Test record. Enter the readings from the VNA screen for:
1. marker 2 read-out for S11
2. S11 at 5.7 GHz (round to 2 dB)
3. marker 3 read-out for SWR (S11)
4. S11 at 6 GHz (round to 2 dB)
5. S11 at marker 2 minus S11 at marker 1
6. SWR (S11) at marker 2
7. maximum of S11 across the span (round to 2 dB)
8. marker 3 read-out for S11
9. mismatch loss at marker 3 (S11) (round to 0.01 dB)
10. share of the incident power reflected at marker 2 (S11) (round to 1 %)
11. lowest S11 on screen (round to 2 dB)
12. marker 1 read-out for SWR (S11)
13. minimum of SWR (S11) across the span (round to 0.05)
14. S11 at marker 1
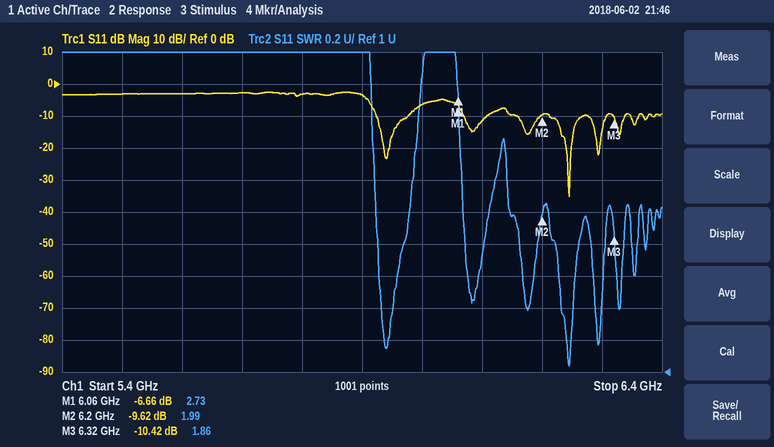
-9.62 dB
-2 dB
1.86
-6 dB
-2.96 dB
1.99
-2 dB
-10.42 dB
0.41 dB
11 %
-36 dB
2.73
1.05
-6.66 dB
